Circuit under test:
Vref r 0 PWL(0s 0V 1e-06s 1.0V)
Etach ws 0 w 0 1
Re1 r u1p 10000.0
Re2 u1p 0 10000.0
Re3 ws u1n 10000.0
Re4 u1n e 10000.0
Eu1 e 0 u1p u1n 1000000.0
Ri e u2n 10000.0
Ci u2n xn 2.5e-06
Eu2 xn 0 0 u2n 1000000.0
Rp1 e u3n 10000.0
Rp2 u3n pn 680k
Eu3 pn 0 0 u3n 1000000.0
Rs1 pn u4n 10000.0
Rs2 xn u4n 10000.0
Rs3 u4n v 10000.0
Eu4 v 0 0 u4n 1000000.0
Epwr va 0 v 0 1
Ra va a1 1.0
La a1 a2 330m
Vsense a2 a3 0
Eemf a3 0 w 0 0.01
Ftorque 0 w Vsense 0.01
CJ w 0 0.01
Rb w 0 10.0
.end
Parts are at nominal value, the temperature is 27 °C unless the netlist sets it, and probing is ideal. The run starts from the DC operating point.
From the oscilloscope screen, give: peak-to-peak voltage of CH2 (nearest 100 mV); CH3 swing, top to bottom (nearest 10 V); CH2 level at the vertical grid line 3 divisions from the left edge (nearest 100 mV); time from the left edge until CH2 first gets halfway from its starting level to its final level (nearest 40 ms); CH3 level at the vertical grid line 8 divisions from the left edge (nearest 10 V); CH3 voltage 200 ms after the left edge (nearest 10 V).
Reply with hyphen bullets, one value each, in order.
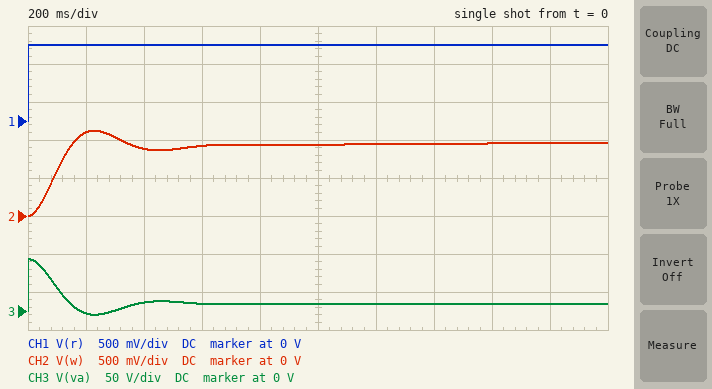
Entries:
- 1.1 V
- 70 V
- 900 mV
- 80 ms
- 10 V
- 0 V
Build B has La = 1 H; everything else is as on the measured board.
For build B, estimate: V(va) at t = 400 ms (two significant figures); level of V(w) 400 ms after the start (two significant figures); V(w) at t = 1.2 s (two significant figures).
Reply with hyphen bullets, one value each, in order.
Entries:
- 6.2 V
- 1.0 V
- 970 mV
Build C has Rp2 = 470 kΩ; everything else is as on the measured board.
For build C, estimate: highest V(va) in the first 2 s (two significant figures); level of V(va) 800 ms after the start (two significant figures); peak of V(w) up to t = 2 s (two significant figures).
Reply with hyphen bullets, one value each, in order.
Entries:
- 47 V
- 9.3 V
- 1.0 V
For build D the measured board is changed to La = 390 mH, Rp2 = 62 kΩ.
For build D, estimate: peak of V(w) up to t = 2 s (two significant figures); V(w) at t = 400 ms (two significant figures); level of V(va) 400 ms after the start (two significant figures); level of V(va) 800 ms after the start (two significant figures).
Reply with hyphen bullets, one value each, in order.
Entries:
- 1.2 V
- 600 mV
- 15 V
- 13 V
